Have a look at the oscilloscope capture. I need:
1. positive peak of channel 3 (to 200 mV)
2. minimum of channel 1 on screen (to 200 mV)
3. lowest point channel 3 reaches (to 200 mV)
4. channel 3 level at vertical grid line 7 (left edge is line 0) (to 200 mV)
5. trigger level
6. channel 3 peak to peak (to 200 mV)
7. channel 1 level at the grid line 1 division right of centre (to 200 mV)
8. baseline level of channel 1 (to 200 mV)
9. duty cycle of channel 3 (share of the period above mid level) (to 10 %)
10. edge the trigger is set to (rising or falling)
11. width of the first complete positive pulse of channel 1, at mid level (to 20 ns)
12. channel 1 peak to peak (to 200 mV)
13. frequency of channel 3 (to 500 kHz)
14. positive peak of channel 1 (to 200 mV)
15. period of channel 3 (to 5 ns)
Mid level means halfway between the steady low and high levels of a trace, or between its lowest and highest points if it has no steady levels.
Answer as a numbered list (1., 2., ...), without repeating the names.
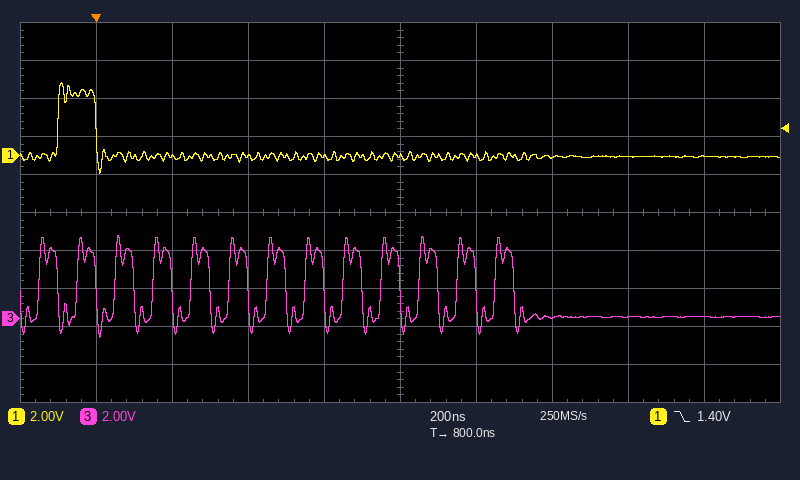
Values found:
1. 4.4 V
2. -1.0 V
3. -1.0 V
4. 0.0 V
5. 1.40 V
6. 5.4 V
7. 0.0 V
8. 0.0 V
9. 50 %
10. falling
11. 100 ns
12. 4.8 V
13. 10.0 MHz
14. 3.8 V
15. 100 ns
